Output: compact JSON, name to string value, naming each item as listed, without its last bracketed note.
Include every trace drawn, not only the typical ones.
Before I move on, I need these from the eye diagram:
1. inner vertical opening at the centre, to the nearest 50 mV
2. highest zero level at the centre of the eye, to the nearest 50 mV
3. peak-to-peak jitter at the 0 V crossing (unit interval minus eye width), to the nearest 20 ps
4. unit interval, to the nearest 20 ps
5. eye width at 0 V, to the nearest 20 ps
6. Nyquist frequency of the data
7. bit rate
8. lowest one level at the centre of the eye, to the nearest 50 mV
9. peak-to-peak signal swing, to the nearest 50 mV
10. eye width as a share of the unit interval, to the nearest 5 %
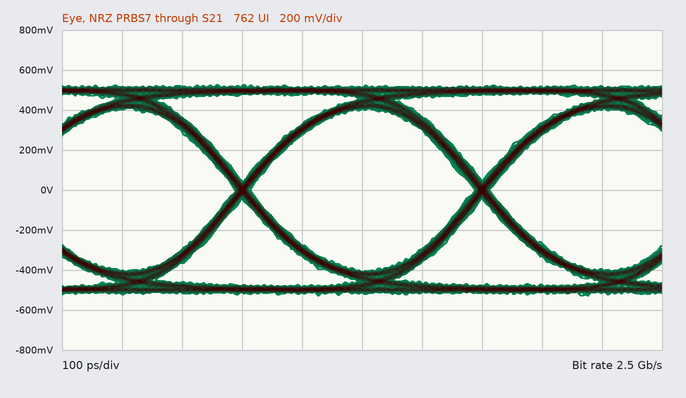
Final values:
{"inner vertical opening at the centre, to the nearest 50 mV": "800 mV", "highest zero level at the centre of the eye, to the nearest 50 mV": "-400 mV", "peak-to-peak jitter at the 0 V crossing (unit interval minus eye width), to the nearest 20 ps": "20 ps", "unit interval, to the nearest 20 ps": "400 ps", "eye width at 0 V, to the nearest 20 ps": "380 ps", "Nyquist frequency of the data": "1.25 GHz", "bit rate": "2.5 Gb/s", "lowest one level at the centre of the eye, to the nearest 50 mV": "400 mV", "peak-to-peak signal swing, to the nearest 50 mV": "1.05 V", "eye width as a share of the unit interval, to the nearest 5 %": "95 %"}
